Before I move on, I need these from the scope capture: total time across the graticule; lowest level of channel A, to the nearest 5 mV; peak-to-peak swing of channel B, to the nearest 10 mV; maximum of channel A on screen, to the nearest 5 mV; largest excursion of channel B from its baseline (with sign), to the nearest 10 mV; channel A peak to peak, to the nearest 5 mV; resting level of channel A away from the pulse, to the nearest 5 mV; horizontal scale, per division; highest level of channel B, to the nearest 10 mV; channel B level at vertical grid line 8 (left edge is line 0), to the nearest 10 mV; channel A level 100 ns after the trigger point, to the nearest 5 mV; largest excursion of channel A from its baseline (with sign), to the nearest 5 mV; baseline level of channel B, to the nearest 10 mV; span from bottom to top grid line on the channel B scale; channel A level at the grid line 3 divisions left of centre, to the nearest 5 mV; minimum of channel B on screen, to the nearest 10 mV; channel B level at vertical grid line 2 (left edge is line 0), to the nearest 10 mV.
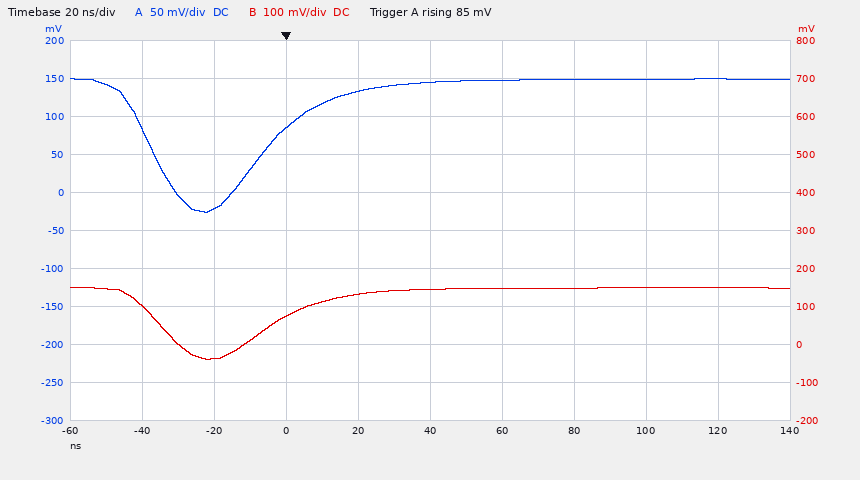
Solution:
200 ns
-25 mV
190 mV
150 mV
-190 mV
175 mV
150 mV
20 ns
150 mV
150 mV
150 mV
-175 mV
150 mV
1 V
-20 mV
-40 mV
-40 mV
